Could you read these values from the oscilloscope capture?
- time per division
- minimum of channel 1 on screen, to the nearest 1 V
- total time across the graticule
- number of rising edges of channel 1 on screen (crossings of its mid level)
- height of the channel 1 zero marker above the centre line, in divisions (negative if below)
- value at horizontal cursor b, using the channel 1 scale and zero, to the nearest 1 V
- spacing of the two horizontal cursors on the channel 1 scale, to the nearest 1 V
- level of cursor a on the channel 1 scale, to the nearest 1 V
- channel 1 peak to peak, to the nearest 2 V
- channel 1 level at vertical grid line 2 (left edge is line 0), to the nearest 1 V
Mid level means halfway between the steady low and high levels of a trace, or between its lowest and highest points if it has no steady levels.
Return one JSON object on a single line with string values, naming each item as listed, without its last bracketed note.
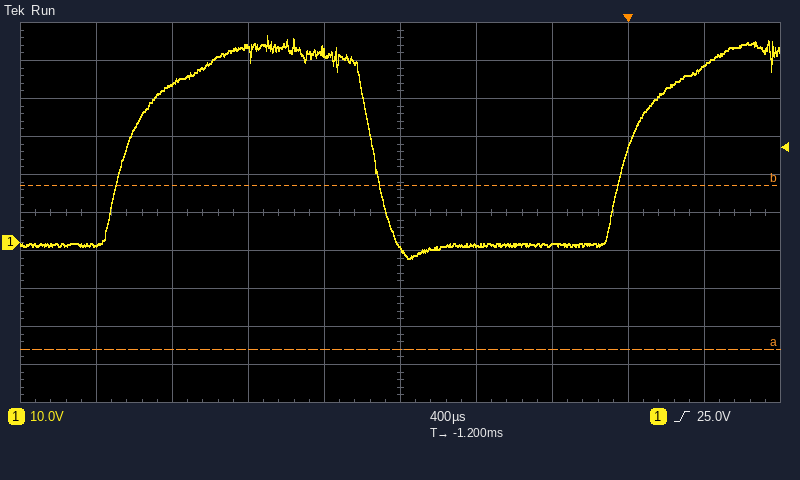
{"time per division": "400 µs", "minimum of channel 1 on screen, to the nearest 1 V": "-4 V", "total time across the graticule": "4 ms", "number of rising edges of channel 1 on screen": "2", "height of the channel 1 zero marker above the centre line, in divisions": "-0.8 div", "value at horizontal cursor b, using the channel 1 scale and zero, to the nearest 1 V": "15 V", "spacing of the two horizontal cursors on the channel 1 scale, to the nearest 1 V": "43 V", "level of cursor a on the channel 1 scale, to the nearest 1 V": "-28 V", "channel 1 peak to peak, to the nearest 2 V": "58 V", "channel 1 level at vertical grid line 2 (left edge is line 0), to the nearest 1 V": "42 V"}
